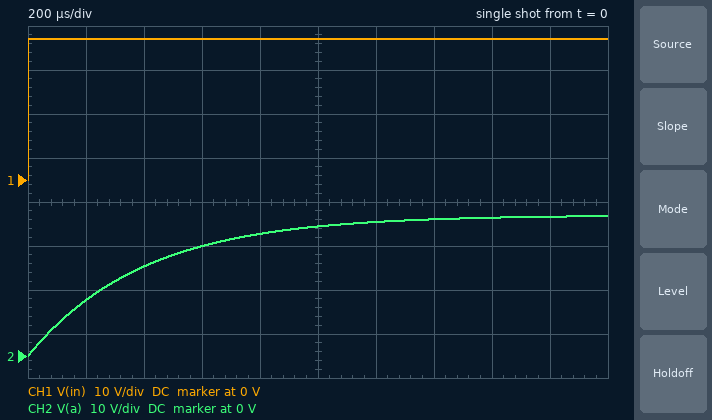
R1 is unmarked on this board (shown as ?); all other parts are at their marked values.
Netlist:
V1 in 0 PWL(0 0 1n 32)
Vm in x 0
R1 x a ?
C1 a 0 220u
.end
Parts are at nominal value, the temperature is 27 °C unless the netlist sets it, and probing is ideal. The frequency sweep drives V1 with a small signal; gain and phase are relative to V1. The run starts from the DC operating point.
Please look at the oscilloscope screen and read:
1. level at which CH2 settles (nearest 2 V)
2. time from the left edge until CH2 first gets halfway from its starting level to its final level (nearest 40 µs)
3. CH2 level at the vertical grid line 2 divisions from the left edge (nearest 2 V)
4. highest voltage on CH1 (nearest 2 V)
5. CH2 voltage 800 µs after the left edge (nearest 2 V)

32 V
280 µs
20 V
32 V
28 V
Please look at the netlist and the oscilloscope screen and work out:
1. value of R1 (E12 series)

1.8 Ω
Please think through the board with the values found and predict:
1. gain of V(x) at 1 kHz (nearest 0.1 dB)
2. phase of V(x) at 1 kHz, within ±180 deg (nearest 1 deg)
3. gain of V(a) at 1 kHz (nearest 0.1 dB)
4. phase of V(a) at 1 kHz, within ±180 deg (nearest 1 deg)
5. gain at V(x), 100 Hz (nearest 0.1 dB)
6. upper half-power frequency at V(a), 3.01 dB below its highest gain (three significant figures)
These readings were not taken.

0 dB
0 deg
-8.6 dB
-68 deg
0 dB
402 Hz
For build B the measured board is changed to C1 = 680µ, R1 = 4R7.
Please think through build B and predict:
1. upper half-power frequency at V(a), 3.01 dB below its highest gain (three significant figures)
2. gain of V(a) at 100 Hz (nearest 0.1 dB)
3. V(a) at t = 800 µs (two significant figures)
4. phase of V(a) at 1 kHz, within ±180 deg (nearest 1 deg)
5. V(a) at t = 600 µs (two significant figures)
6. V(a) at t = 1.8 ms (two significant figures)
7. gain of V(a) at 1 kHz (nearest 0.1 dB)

49.8 Hz
-7.0 dB
7.1 V
-87 deg
5.5 V
14 V
-26.1 dB
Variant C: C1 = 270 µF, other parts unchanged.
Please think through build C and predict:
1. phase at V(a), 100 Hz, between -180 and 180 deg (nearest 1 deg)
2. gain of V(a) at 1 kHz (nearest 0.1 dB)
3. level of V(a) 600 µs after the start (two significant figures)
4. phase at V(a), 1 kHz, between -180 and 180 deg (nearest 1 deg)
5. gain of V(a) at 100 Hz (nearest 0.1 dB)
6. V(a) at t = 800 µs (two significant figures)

-17 deg
-10.1 dB
23 V
-72 deg
-0.4 dB
26 V
